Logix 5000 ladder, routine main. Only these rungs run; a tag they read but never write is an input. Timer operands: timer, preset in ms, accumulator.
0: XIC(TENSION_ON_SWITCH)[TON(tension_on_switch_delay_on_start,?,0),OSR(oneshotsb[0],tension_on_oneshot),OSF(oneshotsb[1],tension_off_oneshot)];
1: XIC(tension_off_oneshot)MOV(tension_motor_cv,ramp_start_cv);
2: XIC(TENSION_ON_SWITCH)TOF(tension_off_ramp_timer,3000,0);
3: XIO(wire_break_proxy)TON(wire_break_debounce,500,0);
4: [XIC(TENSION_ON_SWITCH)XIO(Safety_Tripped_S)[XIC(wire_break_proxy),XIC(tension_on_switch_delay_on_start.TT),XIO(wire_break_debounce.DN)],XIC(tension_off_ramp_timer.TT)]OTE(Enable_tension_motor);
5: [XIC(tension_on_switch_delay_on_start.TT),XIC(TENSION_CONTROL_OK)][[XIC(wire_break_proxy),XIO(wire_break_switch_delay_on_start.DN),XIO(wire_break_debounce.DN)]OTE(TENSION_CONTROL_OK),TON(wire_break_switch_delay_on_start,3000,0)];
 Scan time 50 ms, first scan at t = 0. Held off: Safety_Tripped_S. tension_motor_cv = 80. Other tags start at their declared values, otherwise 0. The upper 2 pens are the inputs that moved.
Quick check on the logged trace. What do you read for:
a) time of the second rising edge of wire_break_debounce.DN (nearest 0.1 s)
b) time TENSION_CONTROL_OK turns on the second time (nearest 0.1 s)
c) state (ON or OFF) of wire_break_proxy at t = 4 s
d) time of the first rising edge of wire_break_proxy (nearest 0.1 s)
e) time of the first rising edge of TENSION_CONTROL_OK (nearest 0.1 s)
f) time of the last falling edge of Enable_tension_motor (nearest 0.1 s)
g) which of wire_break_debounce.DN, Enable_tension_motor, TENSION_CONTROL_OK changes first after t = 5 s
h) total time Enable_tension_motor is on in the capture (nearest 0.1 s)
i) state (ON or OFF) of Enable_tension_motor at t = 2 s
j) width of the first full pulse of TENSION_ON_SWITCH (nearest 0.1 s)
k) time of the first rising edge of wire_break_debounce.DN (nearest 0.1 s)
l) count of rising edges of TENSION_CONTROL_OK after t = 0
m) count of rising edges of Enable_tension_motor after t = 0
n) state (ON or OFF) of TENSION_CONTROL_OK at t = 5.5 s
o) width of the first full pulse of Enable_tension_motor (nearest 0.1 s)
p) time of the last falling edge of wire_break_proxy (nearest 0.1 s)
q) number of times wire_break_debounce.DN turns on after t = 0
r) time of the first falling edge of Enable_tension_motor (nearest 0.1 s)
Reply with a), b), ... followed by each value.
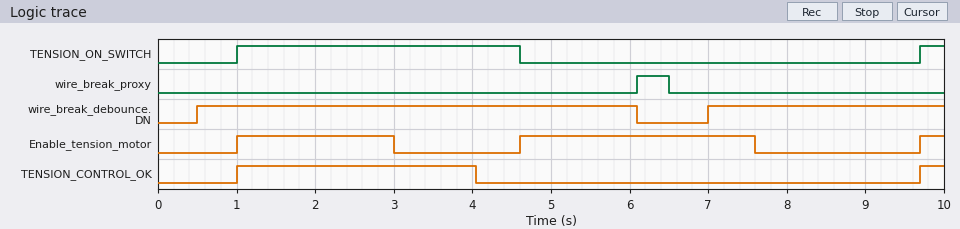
a) 7.0 s
b) 9.7 s
c) OFF
d) 6.1 s
e) 1.0 s
f) 7.6 s
g) wire_break_debounce.DN
h) 5.3 s
i) ON
j) 3.6 s
k) 0.5 s
l) 2
m) 3
n) OFF
o) 2.0 s
p) 6.5 s
q) 2
r) 3.0 s
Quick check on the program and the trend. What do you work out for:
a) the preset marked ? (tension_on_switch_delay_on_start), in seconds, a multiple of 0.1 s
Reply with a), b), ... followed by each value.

a) 2.0 s
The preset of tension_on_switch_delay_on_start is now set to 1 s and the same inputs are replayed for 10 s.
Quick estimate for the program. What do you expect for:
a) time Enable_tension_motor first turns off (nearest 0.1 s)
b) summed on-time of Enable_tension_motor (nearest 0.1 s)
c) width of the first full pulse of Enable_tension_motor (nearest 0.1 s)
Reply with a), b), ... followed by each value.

a) 2.0 s
b) 4.3 s
c) 1.0 s
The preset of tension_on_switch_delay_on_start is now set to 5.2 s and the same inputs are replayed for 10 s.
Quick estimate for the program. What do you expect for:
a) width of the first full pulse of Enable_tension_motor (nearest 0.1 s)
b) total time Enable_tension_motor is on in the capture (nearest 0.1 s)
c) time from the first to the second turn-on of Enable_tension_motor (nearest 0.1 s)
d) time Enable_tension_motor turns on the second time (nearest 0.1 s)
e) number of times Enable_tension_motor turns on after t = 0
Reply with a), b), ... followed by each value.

a) 6.6 s
b) 6.9 s
c) 8.7 s
d) 9.7 s
e) 2
